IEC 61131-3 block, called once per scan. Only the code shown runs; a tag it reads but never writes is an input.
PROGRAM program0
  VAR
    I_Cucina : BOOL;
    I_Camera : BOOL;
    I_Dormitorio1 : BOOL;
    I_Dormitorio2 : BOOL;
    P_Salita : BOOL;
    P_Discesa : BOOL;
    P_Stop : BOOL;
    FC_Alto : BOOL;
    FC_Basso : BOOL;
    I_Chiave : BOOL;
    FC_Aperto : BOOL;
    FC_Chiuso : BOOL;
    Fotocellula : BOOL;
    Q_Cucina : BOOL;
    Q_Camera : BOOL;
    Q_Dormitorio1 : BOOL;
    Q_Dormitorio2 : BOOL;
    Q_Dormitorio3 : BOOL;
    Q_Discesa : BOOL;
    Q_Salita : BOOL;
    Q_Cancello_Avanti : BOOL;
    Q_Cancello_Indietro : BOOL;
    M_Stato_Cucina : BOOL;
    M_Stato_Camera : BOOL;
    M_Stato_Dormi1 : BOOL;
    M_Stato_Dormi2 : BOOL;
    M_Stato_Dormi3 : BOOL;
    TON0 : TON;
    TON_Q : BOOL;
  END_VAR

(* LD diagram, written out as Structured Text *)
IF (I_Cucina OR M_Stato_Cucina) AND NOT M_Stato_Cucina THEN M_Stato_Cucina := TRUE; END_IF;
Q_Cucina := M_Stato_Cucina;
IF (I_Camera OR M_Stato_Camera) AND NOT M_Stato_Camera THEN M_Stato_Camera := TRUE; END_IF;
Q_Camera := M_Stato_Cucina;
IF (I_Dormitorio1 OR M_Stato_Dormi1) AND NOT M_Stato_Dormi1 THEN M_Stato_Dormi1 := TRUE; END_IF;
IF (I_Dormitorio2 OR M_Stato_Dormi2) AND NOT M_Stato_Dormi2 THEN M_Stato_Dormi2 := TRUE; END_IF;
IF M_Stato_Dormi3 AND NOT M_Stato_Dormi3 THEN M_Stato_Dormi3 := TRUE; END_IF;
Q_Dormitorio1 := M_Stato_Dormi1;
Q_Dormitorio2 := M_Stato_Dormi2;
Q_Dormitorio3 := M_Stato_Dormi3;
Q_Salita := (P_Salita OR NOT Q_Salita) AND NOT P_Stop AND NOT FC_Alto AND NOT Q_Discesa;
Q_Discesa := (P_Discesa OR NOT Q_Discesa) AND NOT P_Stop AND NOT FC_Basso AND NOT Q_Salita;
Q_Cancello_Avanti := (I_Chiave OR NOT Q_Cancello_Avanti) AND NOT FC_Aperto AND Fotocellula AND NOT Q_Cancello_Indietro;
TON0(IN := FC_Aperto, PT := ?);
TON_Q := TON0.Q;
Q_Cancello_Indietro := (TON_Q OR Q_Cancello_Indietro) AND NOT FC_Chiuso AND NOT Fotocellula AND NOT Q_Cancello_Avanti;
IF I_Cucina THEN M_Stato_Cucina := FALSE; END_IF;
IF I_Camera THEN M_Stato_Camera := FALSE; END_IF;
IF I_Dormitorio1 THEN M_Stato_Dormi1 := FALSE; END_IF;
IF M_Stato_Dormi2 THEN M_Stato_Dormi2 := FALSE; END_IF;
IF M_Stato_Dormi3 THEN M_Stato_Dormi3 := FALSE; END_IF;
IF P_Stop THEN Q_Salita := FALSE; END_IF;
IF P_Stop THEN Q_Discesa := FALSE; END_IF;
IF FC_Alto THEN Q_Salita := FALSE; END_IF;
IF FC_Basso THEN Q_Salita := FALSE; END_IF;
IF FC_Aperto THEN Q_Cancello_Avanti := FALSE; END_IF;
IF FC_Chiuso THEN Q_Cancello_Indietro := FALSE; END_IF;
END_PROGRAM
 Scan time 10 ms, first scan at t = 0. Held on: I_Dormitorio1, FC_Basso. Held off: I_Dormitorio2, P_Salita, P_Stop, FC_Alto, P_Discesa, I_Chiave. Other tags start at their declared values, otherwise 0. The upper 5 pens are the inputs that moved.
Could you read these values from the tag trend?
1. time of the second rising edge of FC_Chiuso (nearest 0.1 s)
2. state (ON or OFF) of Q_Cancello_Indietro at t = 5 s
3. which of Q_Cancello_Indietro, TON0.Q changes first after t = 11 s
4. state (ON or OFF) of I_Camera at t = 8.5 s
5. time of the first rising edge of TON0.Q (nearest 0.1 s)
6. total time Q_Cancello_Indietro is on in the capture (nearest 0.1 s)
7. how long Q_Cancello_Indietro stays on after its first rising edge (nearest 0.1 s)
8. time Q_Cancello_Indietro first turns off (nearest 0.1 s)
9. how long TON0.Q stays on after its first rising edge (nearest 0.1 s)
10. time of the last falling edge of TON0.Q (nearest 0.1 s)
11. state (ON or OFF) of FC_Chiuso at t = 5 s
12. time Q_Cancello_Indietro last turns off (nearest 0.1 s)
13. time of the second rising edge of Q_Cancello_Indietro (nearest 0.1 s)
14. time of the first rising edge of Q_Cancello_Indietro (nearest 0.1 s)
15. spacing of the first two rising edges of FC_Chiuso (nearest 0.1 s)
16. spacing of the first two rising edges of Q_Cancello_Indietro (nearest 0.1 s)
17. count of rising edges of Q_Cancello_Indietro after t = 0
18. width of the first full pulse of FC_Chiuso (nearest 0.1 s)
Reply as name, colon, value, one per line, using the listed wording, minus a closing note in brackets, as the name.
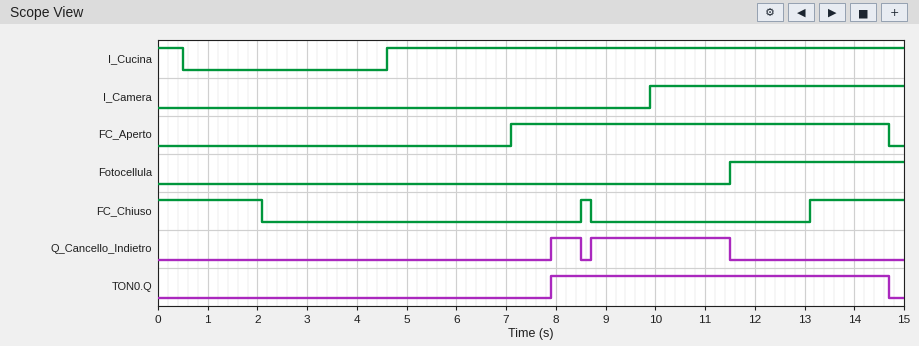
time of the second rising edge of FC_Chiuso: 13.1 s
state (ON or OFF) of Q_Cancello_Indietro at t = 5 s: OFF
which of Q_Cancello_Indietro, TON0.Q changes first after t = 11 s: Q_Cancello_Indietro
state (ON or OFF) of I_Camera at t = 8.5 s: OFF
time of the first rising edge of TON0.Q: 7.9 s
total time Q_Cancello_Indietro is on in the capture: 3.4 s
how long Q_Cancello_Indietro stays on after its first rising edge: 0.6 s
time Q_Cancello_Indietro first turns off: 8.5 s
how long TON0.Q stays on after its first rising edge: 6.8 s
time of the last falling edge of TON0.Q: 14.7 s
state (ON or OFF) of FC_Chiuso at t = 5 s: OFF
time Q_Cancello_Indietro last turns off: 11.5 s
time of the second rising edge of Q_Cancello_Indietro: 8.7 s
time of the first rising edge of Q_Cancello_Indietro: 7.9 s
spacing of the first two rising edges of FC_Chiuso: 4.6 s
spacing of the first two rising edges of Q_Cancello_Indietro: 0.8 s
count of rising edges of Q_Cancello_Indietro after t = 0: 2
width of the first full pulse of FC_Chiuso: 0.2 s
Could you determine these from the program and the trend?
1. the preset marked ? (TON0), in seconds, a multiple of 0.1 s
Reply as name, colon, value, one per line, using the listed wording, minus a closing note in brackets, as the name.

the preset marked ? (TON0), in seconds, a multiple of 0.1 s: 0.8 s
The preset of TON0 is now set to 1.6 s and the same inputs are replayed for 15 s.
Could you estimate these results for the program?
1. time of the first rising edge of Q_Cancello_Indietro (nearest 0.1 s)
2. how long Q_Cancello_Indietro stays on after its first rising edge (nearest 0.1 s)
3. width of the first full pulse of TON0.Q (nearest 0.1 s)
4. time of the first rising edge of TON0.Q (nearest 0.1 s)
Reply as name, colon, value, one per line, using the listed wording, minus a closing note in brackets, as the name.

time of the first rising edge of Q_Cancello_Indietro: 8.7 s
how long Q_Cancello_Indietro stays on after its first rising edge: 2.8 s
width of the first full pulse of TON0.Q: 6.0 s
time of the first rising edge of TON0.Q: 8.7 s
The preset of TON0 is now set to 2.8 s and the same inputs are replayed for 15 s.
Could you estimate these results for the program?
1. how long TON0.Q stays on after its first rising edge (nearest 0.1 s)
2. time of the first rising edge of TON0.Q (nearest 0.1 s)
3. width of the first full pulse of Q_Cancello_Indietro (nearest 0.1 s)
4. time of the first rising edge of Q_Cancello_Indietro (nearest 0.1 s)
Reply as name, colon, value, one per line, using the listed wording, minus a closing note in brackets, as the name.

how long TON0.Q stays on after its first rising edge: 4.8 s
time of the first rising edge of TON0.Q: 9.9 s
width of the first full pulse of Q_Cancello_Indietro: 1.6 s
time of the first rising edge of Q_Cancello_Indietro: 9.9 s
